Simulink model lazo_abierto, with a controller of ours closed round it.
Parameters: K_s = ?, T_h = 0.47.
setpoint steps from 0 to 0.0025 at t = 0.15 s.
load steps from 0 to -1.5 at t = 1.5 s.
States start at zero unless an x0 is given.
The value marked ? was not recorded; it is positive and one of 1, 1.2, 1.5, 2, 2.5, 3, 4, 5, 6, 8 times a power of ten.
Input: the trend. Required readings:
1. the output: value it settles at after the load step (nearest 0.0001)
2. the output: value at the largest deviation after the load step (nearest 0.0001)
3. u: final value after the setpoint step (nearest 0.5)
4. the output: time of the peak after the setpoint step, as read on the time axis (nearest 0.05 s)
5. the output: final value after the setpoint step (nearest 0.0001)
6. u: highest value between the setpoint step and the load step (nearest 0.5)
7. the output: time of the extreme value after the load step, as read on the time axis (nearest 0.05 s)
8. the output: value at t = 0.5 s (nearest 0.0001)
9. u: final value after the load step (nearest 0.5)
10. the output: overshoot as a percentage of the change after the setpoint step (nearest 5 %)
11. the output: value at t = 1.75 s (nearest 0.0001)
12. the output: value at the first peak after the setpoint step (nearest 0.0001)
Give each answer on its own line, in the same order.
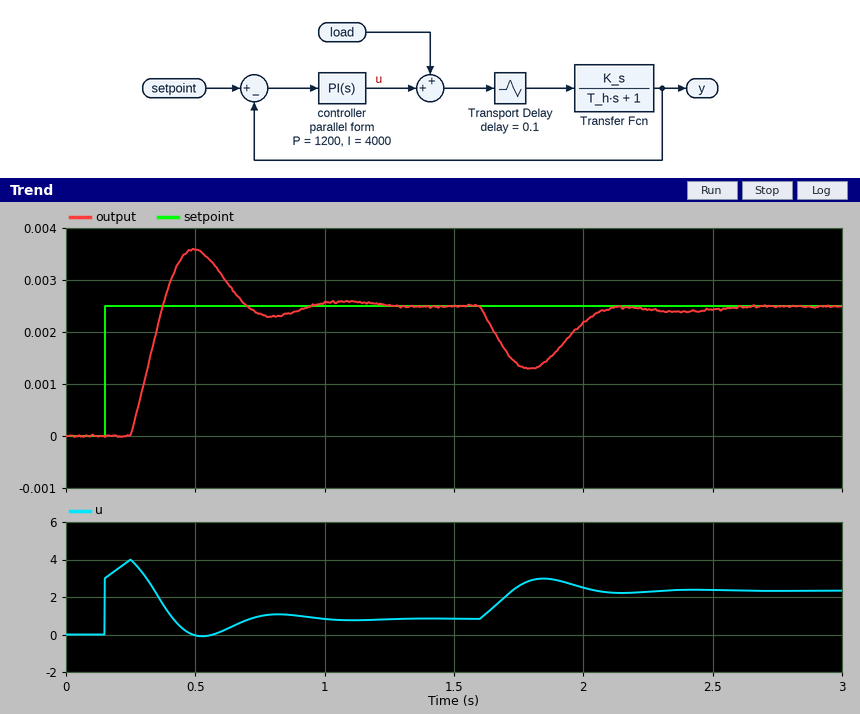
0.0025
0.0013
1.0
0.50 s
0.0025
4.0
1.80 s
0.0036
2.5
45 %
0.0014
0.0036
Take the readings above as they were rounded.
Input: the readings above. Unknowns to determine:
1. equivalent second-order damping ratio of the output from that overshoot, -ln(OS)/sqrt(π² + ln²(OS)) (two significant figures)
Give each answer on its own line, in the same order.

0.25
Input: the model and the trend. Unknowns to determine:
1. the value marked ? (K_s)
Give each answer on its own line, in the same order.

0.003
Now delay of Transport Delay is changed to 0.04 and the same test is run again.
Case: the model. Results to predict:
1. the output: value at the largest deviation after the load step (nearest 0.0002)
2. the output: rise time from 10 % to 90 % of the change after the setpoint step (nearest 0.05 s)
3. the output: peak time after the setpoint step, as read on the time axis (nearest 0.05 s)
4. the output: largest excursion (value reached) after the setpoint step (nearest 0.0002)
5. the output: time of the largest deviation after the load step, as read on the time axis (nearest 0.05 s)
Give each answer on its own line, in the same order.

0.0016
0.15 s
0.55 s
0.0026
1.70 s
